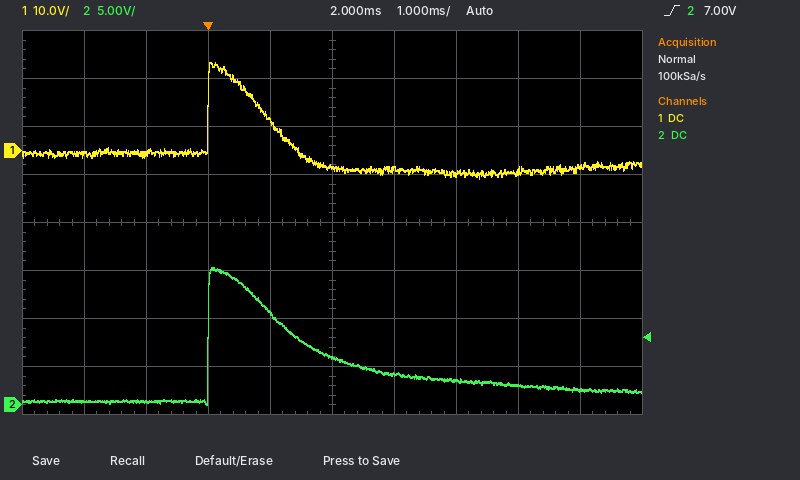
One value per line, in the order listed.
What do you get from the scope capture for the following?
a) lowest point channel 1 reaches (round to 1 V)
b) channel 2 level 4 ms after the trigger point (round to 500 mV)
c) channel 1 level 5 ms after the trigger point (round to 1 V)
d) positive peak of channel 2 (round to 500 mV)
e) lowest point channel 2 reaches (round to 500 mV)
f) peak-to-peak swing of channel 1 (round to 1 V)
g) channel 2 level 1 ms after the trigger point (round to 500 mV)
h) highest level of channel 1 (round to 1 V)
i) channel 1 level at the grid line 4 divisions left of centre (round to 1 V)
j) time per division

-6 V
2.5 V
-4 V
14.5 V
0.0 V
24 V
9.5 V
18 V
-1 V
1 ms
